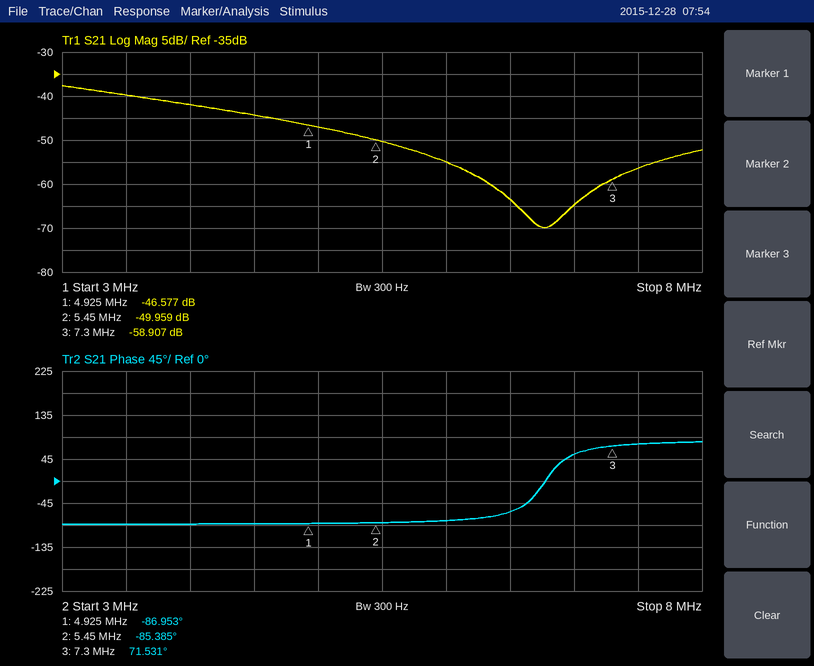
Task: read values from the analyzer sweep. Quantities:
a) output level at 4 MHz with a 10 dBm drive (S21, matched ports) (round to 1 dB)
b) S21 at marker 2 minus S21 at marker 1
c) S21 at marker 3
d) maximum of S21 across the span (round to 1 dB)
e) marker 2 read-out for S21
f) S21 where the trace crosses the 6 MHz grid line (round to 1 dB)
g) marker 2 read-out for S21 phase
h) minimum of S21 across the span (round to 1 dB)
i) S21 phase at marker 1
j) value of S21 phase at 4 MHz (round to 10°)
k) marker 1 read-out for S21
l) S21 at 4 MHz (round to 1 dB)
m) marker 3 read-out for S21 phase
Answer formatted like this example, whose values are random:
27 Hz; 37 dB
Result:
-32 dBm; -3.382 dB; -58.907 dB; -38 dB; -49.959 dB; -55 dB; -85.385°; -70 dB; -86.953°; -90°; -46.577 dB; -42 dB; 71.531°
